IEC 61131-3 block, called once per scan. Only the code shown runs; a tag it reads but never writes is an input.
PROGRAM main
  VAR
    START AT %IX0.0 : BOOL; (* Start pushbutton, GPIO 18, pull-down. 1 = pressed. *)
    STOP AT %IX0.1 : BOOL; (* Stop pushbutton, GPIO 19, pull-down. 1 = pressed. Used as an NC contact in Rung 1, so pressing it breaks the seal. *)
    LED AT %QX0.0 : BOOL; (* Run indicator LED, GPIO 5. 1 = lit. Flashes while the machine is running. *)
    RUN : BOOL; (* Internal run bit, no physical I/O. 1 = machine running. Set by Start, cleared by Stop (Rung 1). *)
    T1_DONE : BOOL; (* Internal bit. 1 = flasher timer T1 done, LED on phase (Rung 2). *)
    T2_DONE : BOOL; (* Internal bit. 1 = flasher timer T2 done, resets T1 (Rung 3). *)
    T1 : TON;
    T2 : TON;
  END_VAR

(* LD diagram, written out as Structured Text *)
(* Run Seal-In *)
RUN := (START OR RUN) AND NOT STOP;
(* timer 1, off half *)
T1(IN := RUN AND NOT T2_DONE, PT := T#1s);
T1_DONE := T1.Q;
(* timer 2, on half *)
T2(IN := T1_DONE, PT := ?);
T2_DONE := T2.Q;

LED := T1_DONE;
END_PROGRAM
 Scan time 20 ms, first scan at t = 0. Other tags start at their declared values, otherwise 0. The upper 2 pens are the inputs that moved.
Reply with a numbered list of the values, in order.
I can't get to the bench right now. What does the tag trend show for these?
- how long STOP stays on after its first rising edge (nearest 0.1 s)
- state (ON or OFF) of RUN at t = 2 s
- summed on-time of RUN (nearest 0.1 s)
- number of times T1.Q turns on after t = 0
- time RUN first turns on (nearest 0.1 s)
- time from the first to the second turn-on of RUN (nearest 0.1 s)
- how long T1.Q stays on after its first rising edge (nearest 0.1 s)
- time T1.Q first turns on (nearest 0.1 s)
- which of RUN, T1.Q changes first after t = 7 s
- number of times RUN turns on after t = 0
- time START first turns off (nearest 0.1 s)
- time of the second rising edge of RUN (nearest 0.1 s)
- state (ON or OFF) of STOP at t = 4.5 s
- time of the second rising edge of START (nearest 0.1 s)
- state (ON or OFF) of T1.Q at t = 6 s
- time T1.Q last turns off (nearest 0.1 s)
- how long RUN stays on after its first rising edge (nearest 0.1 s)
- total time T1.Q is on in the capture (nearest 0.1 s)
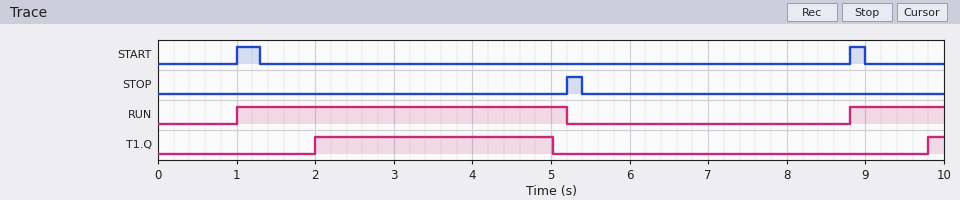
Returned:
1. 0.2 s
2. ON
3. 5.4 s
4. 2
5. 1.0 s
6. 7.8 s
7. 3.0 s
8. 2.0 s
9. RUN
10. 2
11. 1.3 s
12. 8.8 s
13. OFF
14. 8.8 s
15. OFF
16. 5.0 s
17. 4.2 s
18. 3.2 s
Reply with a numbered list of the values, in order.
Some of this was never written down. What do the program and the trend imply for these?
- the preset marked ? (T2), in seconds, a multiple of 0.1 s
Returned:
1. 3.0 s
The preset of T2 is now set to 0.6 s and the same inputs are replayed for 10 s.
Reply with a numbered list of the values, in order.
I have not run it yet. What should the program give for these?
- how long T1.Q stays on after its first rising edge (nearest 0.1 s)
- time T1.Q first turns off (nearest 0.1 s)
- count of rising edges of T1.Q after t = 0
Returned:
1. 0.6 s
2. 2.6 s
3. 3
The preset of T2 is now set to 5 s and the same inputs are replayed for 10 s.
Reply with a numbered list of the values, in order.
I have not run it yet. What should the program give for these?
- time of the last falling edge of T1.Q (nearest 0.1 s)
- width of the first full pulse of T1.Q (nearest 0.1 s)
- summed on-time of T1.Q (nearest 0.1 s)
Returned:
1. 5.2 s
2. 3.2 s
3. 3.4 s
